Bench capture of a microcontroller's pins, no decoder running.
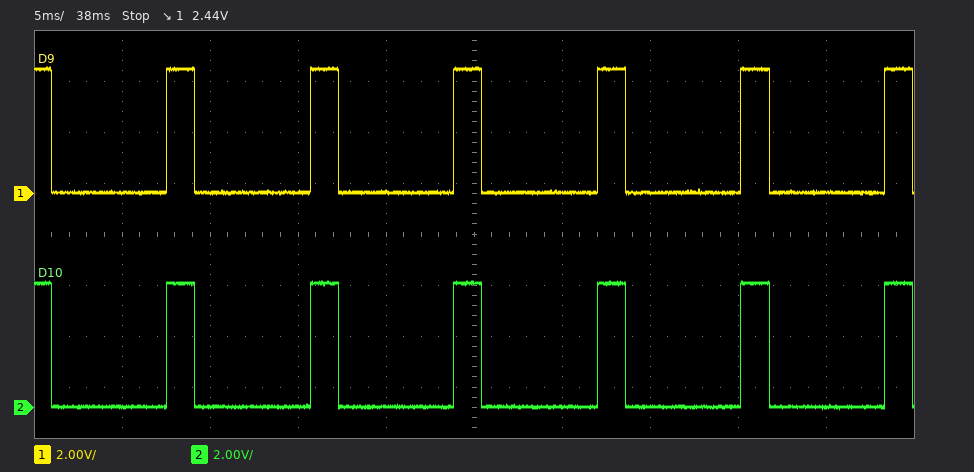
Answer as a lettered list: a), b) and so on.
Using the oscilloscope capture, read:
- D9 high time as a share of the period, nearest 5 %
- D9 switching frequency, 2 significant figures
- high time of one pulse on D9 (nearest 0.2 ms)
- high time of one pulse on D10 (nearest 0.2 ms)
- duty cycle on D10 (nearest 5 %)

a) 20 %
b) 120 Hz
c) 1.6 ms
d) 1.6 ms
e) 20 %
